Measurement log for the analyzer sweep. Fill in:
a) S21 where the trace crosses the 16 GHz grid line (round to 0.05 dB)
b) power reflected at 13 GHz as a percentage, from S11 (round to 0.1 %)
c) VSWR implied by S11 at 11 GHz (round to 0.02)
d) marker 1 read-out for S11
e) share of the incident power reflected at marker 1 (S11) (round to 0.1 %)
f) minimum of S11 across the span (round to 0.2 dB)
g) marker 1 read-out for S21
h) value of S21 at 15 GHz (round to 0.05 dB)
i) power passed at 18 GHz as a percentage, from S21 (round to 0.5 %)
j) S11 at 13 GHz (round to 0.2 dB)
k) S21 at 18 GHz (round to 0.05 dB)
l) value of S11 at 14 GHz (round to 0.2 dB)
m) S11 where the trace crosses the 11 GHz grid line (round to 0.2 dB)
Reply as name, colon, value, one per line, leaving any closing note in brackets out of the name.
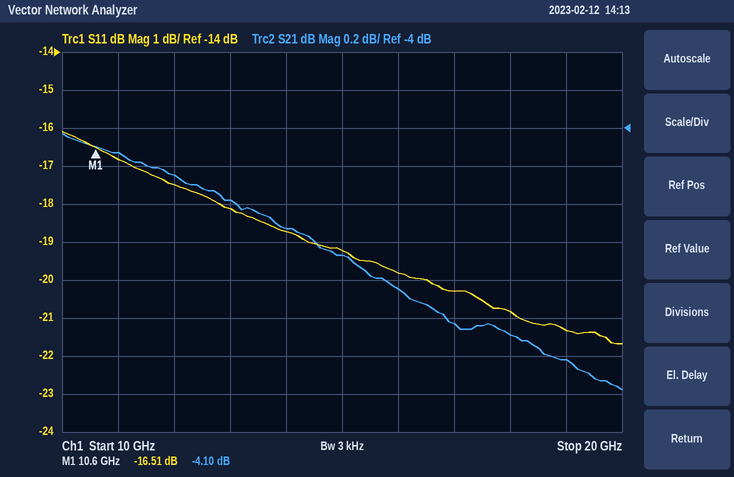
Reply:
S21 where the trace crosses the 16 GHz grid line: -4.85 dB
power reflected at 13 GHz as a percentage, from S11: 1.5 %
VSWR implied by S11 at 11 GHz: 1.34
marker 1 read-out for S11: -16.51 dB
share of the incident power reflected at marker 1 (S11): 2.2 %
minimum of S11 across the span: -21.6 dB
marker 1 read-out for S21: -4.10 dB
value of S21 at 15 GHz: -4.65 dB
power passed at 18 GHz as a percentage, from S21: 31.0 %
S11 at 13 GHz: -18.2 dB
S21 at 18 GHz: -5.10 dB
value of S11 at 14 GHz: -18.8 dB
S11 where the trace crosses the 11 GHz grid line: -16.8 dB
